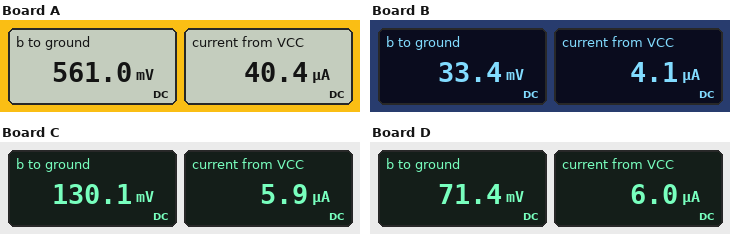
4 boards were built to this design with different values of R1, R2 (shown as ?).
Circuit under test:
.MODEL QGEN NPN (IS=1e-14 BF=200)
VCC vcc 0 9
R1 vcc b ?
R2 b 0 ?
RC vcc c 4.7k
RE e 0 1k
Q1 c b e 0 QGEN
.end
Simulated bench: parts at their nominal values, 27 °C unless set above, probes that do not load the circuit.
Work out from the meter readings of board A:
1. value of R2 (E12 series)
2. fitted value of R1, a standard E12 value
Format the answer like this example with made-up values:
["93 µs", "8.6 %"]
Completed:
["22 kΩ", "330 kΩ"]
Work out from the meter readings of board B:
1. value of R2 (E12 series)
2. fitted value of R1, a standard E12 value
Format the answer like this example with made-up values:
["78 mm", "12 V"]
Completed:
["8.2 kΩ", "2.2 MΩ"]
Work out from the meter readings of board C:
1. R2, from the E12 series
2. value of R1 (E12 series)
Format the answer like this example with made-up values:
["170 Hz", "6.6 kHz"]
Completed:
["22 kΩ", "1.5 MΩ"]
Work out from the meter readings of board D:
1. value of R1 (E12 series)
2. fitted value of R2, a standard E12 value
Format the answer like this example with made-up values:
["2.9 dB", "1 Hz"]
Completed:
["1.5 MΩ", "12 kΩ"]
